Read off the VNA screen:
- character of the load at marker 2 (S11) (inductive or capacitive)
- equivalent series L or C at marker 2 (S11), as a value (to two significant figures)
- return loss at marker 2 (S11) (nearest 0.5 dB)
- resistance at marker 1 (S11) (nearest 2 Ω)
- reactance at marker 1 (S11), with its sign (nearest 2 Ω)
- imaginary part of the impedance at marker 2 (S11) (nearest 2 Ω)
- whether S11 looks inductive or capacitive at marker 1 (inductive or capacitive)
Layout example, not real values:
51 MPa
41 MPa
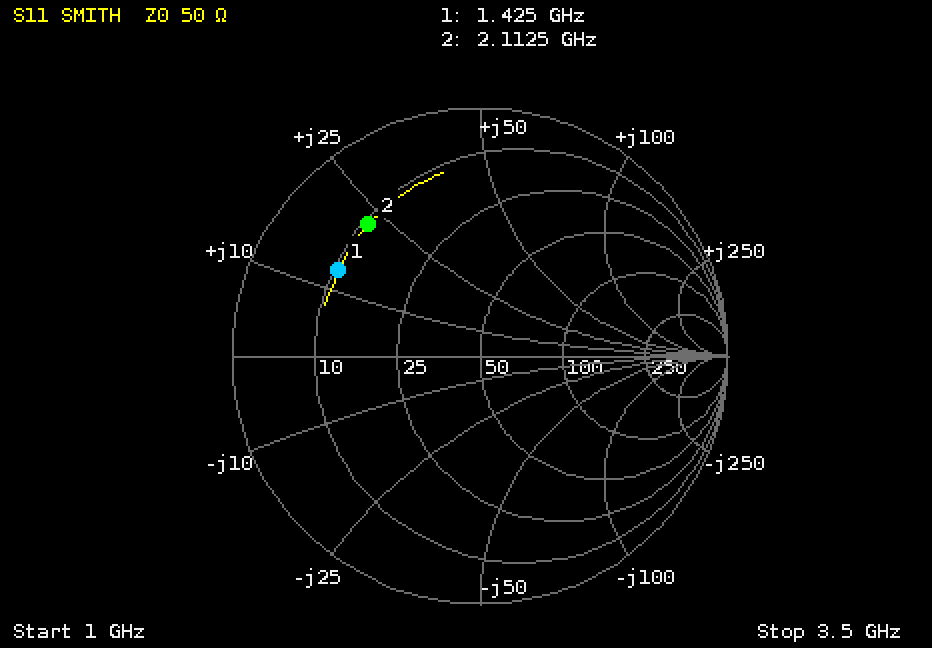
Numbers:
inductive
1.7 nH
3.0 dB
10 Ω
+14 Ω
+22 Ω
inductive
